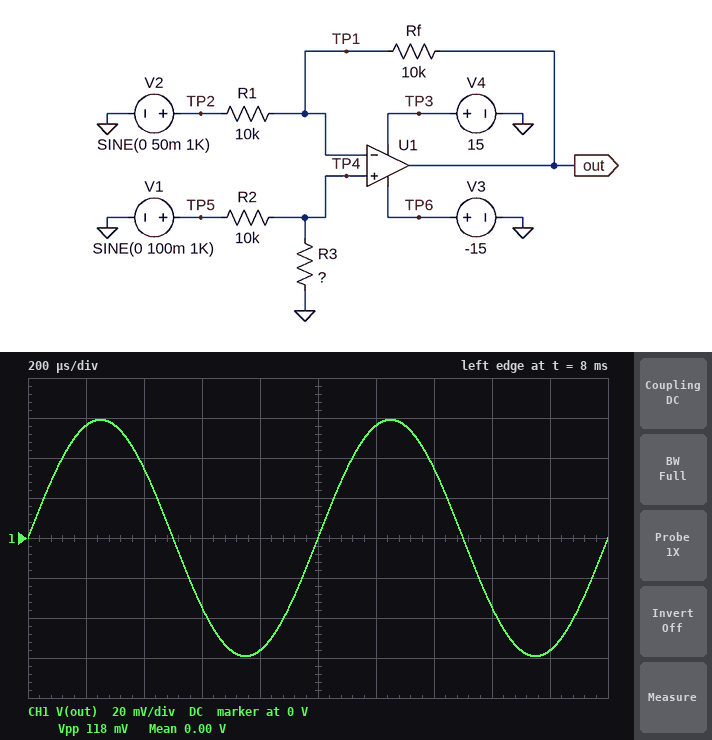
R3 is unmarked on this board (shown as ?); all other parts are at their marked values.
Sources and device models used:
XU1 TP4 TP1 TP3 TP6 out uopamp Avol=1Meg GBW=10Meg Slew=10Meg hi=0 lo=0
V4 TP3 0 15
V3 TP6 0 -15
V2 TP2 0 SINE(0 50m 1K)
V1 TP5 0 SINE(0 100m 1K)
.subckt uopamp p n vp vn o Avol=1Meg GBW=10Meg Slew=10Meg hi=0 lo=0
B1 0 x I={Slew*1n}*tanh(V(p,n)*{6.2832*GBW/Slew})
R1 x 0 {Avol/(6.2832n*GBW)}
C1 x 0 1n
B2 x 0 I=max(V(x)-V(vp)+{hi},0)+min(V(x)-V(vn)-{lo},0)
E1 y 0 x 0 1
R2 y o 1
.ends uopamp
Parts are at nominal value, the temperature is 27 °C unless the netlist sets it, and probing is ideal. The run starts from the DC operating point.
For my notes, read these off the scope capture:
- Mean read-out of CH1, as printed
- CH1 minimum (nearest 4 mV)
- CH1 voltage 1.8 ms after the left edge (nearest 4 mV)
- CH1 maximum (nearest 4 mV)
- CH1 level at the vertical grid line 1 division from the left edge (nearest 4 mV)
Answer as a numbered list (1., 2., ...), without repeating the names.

1. 0.00 V
2. -60 mV
3. -56 mV
4. 60 mV
5. 56 mV
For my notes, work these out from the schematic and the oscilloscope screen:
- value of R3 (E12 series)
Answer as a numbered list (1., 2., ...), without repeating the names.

1. 12 kΩ
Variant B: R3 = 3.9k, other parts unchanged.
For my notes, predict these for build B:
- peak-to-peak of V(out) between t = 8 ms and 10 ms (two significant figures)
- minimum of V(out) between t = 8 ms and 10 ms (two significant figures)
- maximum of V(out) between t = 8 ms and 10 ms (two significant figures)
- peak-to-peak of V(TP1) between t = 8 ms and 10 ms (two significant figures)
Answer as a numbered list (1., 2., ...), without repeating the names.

1. 12 mV
2. -6.1 mV
3. 6.1 mV
4. 56 mV
